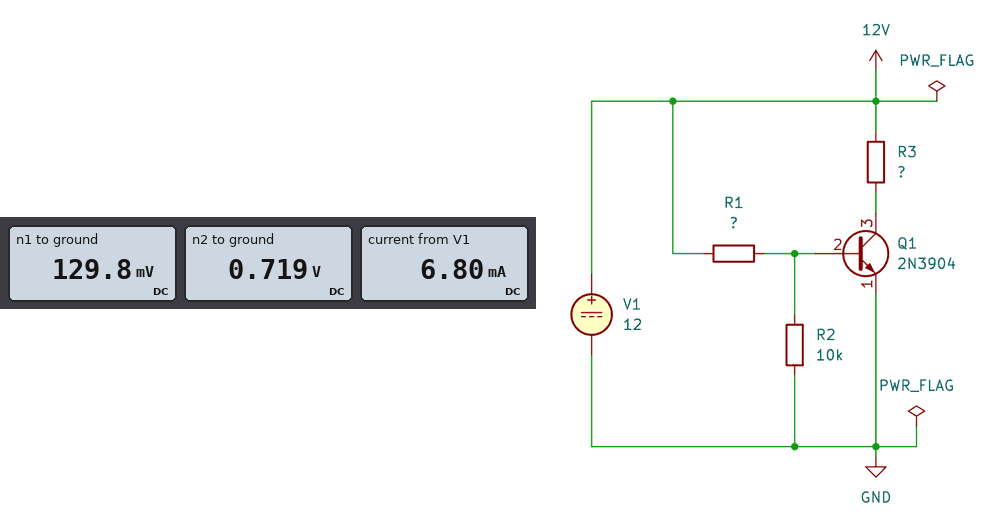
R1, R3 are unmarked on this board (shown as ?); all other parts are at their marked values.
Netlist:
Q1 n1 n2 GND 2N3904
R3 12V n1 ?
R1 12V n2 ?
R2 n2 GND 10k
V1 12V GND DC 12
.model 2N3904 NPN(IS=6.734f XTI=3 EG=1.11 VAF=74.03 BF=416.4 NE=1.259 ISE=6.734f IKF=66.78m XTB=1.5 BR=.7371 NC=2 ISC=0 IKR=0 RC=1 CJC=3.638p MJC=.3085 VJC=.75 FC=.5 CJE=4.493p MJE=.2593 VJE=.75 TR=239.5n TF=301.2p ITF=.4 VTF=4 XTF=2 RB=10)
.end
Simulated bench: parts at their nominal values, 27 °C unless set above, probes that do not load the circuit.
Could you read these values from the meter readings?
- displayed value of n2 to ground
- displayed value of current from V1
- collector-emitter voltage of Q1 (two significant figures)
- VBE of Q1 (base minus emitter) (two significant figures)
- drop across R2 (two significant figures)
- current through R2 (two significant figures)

0.719 V
6.80 mA
130 mV
720 mV
720 mV
72 µA
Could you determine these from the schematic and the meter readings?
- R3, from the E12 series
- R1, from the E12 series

1.8 kΩ
56 kΩ
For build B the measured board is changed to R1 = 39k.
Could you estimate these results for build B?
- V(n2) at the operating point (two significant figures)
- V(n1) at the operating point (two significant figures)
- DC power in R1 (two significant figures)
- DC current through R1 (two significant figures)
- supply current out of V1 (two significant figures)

720 mV
110 mV
3.3 mW
290 µA
6.9 mA
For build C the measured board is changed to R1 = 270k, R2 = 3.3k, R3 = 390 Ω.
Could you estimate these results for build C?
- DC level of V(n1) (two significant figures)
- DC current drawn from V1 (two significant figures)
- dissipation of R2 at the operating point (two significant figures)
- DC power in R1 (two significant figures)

12 V
44 µA
6.4 µW
520 µW
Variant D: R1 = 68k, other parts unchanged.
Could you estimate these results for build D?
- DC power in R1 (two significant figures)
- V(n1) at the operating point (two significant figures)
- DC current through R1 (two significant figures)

1.9 mW
140 mV
170 µA
